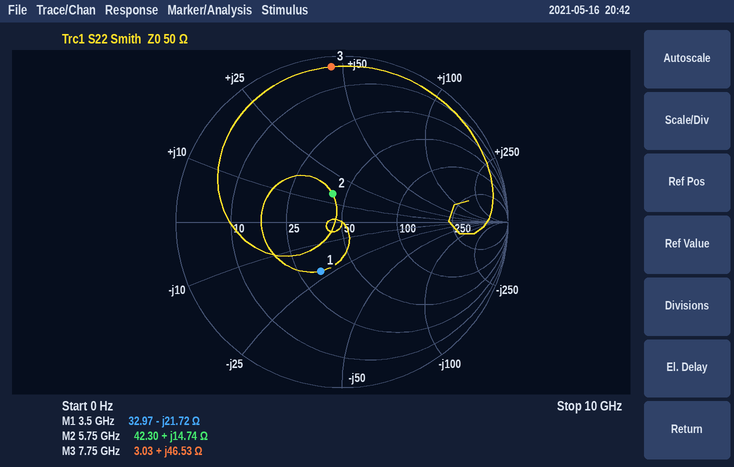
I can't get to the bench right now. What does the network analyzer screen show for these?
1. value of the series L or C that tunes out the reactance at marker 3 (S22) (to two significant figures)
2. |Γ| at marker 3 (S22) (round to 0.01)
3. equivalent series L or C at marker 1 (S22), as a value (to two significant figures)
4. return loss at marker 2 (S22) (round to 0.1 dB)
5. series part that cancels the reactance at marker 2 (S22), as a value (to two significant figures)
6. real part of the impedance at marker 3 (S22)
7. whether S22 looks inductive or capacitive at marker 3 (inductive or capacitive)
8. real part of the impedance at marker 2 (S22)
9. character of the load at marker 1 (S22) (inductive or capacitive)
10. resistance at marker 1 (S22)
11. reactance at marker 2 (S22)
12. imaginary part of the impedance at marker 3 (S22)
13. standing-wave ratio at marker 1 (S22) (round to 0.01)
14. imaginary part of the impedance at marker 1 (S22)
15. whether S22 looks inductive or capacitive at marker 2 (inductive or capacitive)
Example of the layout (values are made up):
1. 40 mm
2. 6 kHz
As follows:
1. 440 fF
2. 0.94
3. 2.1 pF
4. 15.0 dB
5. 1.9 pF
6. 3.03 Ω
7. inductive
8. 42.30 Ω
9. capacitive
10. 32.97 Ω
11. +14.74 Ω
12. +46.53 Ω
13. 1.95
14. -21.72 Ω
15. inductive
